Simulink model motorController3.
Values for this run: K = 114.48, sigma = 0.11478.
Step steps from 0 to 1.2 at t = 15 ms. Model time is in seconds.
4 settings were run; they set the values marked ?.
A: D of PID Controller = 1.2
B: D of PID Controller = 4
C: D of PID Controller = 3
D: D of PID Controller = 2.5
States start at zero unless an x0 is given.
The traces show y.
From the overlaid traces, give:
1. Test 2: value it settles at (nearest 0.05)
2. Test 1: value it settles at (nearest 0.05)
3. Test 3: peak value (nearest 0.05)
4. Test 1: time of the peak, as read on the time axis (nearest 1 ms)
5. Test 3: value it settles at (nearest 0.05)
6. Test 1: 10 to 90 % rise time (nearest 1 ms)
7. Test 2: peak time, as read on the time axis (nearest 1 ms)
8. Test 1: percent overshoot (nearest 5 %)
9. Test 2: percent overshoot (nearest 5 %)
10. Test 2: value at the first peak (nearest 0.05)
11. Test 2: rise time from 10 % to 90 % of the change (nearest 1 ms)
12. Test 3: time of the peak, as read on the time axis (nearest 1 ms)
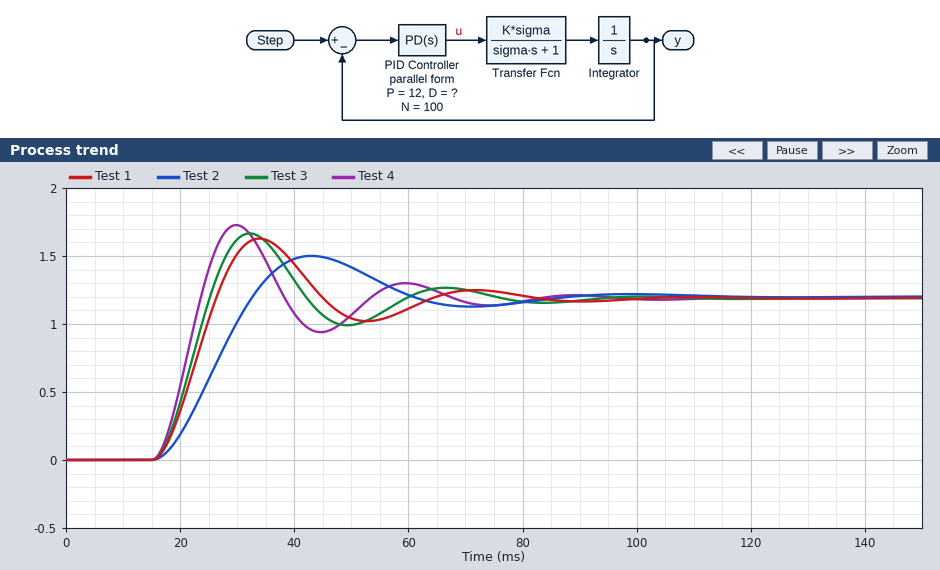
1.20
1.20
1.65
34 ms
1.20
8 ms
43 ms
35 %
25 %
1.50
12 ms
32 ms
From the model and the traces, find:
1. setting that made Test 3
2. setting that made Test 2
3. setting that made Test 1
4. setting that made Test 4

C
A
D
B
